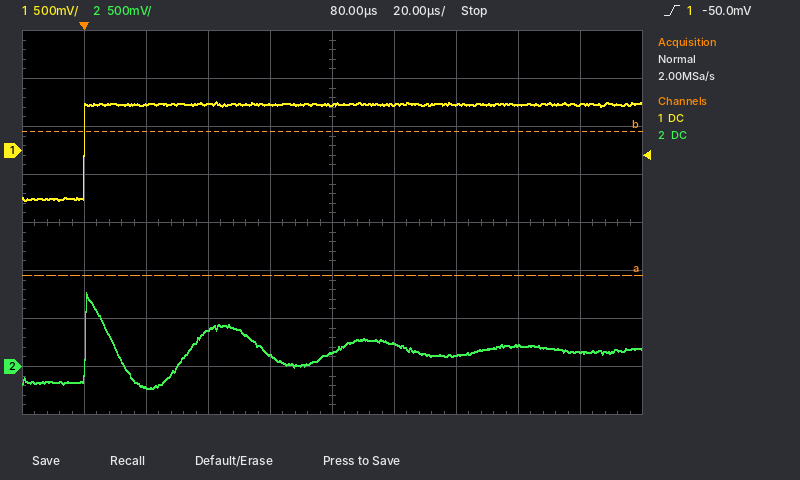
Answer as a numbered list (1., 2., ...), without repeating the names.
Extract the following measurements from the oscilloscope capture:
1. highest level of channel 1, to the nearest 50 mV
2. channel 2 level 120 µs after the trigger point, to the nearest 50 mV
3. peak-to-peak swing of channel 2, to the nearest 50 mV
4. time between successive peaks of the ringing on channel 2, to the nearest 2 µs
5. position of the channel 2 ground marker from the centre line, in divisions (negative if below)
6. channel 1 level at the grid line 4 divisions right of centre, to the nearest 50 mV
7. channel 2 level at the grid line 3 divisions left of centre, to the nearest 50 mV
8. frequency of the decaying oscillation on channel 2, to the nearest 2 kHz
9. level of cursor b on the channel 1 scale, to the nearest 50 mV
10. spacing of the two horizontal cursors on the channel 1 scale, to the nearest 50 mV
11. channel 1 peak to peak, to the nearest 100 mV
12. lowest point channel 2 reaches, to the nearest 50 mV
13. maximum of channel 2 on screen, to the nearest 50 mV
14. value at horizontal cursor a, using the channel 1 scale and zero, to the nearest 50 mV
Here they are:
1. 500 mV
2. 100 mV
3. 1.00 V
4. 44 µs
5. -3.0 div
6. 500 mV
7. -200 mV
8. 22 kHz
9. 200 mV
10. 1.50 V
11. 1.00 V
12. -250 mV
13. 750 mV
14. -1.30 V
